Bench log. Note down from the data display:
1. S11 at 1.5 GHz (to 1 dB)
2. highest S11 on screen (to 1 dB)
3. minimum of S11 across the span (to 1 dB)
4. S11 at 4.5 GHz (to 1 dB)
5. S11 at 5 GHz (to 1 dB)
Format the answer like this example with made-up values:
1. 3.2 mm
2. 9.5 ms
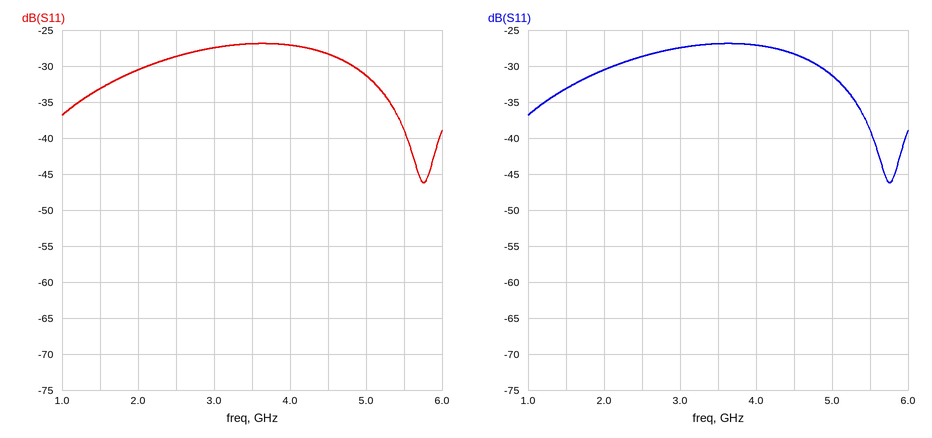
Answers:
1. -33 dB
2. -27 dB
3. -46 dB
4. -28 dB
5. -31 dB
